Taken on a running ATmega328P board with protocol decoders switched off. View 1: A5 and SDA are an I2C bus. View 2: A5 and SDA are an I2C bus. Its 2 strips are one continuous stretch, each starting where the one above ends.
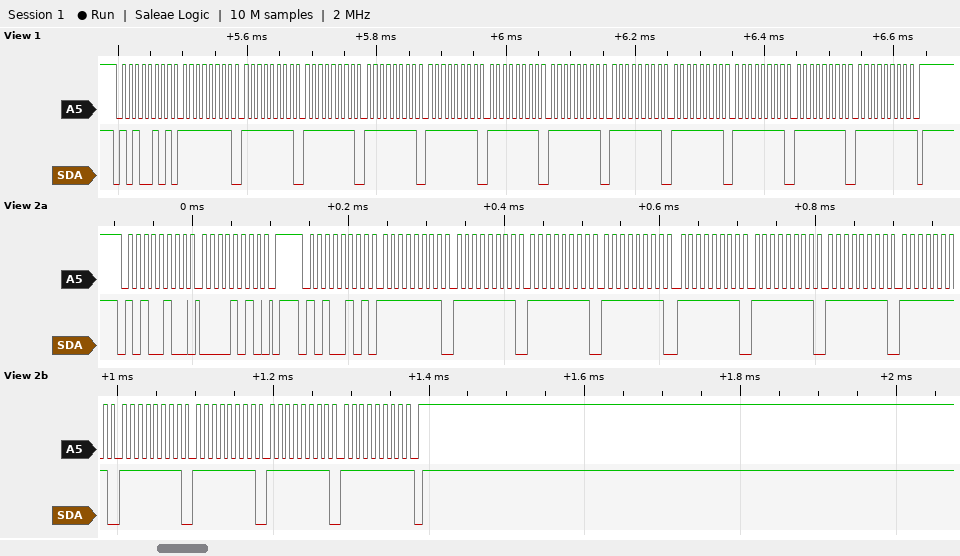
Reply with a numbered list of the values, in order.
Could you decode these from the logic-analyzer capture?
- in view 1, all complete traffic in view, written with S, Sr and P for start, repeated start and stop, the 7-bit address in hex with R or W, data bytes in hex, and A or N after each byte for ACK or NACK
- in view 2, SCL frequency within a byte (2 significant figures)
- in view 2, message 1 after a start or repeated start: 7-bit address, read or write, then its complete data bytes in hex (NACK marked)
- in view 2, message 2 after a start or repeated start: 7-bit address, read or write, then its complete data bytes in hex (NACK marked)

1. S 52R A FF A FF A FF A FF A FF A FF A FF A FF A FF A FF A FF A FF N P
2. 100 kHz
3. 0x52 write: 0A
4. 0x52 read: FF FF FF FF FF FF FF FF FF FF FF FF NACK
